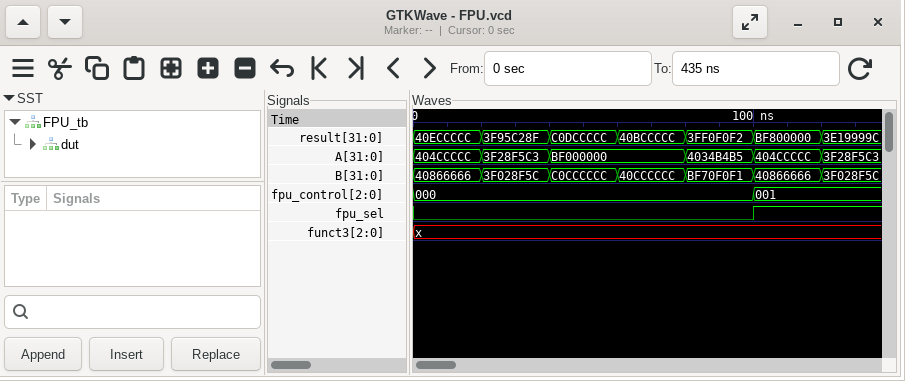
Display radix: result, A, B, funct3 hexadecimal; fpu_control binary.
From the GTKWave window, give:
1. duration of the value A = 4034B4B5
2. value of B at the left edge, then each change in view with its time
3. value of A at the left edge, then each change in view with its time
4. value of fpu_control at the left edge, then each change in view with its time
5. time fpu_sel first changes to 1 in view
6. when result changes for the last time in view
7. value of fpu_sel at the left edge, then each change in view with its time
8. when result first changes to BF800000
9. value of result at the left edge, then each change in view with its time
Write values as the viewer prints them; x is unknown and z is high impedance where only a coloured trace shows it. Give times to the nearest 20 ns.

20 ns
40866666, 3F028F5C at 20 ns, C0CCCCCC at 40 ns, 40CCCCCC at 60 ns, BF70F0F1 at 80 ns, 40866666 at 100 ns, 3F028F5C at 120 ns
404CCCCC, 3F28F5C3 at 20 ns, BF000000 at 40 ns, 4034B4B5 at 80 ns, 404CCCCC at 100 ns, 3F28F5C3 at 120 ns
000, 001 at 100 ns
100 ns
120 ns
0, 1 at 100 ns
100 ns
40ECCCCC, 3F95C28F at 20 ns, C0DCCCCC at 40 ns, 40BCCCCC at 60 ns, 3FF0F0F2 at 80 ns, BF800000 at 100 ns, 3E19999C at 120 ns
